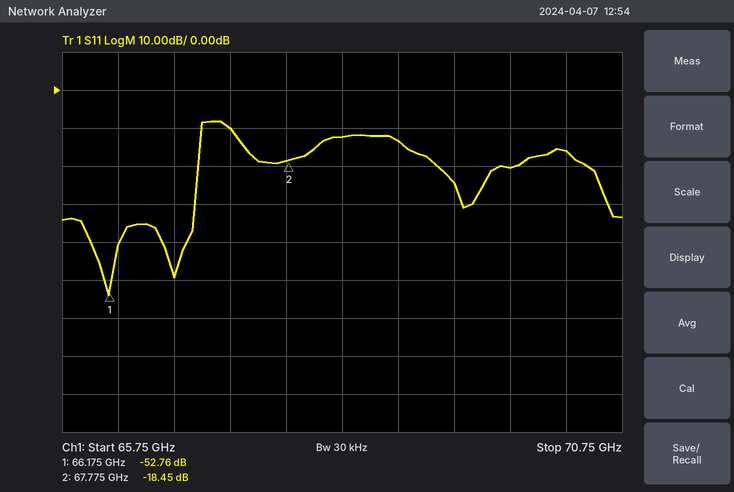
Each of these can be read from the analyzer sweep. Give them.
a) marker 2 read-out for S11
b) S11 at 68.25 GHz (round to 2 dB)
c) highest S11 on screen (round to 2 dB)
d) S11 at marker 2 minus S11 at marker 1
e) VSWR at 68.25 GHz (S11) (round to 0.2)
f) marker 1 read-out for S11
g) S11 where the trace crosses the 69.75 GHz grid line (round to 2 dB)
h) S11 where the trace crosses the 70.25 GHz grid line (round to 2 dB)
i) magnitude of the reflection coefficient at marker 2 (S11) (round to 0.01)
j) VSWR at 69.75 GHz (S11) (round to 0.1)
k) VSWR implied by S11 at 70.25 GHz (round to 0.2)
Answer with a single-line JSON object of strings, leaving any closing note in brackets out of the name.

{"marker 2 read-out for S11": "-18.45 dB", "S11 at 68.25 GHz": "-12 dB", "highest S11 on screen": "-8 dB", "S11 at marker 2 minus S11 at marker 1": "34.31 dB", "VSWR at 68.25 GHz (S11)": "1.6", "marker 1 read-out for S11": "-52.76 dB", "S11 where the trace crosses the 69.75 GHz grid line": "-20 dB", "S11 where the trace crosses the 70.25 GHz grid line": "-16 dB", "magnitude of the reflection coefficient at marker 2 (S11)": "0.12", "VSWR at 69.75 GHz (S11)": "1.2", "VSWR implied by S11 at 70.25 GHz": "1.4"}
